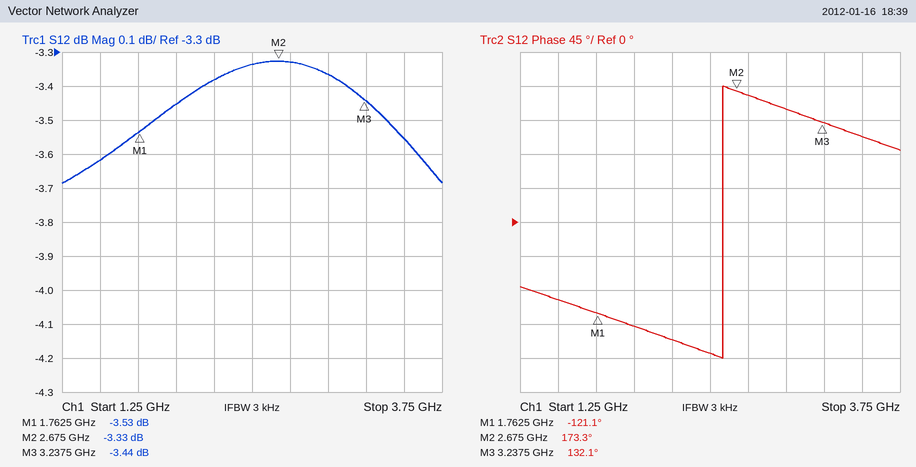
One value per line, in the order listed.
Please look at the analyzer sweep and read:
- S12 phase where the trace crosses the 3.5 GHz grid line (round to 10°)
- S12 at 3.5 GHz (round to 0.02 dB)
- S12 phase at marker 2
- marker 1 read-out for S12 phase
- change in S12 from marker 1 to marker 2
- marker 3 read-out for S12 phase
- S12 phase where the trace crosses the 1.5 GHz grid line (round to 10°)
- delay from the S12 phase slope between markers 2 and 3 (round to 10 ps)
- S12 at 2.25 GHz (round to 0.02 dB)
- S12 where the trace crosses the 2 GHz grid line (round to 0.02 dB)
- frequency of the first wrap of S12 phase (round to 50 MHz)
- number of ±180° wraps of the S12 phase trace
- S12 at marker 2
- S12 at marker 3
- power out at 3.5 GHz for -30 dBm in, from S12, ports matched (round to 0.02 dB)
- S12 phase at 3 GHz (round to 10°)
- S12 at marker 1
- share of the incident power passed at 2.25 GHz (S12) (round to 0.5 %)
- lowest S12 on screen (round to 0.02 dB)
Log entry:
110°
-3.56 dB
173.3°
-121.1°
0.20 dB
132.1°
-100°
200 ps
-3.38 dB
-3.46 dB
2.60 GHz
1
-3.33 dB
-3.44 dB
-33.56 dBm
150°
-3.53 dB
46.0 %
-3.68 dB
